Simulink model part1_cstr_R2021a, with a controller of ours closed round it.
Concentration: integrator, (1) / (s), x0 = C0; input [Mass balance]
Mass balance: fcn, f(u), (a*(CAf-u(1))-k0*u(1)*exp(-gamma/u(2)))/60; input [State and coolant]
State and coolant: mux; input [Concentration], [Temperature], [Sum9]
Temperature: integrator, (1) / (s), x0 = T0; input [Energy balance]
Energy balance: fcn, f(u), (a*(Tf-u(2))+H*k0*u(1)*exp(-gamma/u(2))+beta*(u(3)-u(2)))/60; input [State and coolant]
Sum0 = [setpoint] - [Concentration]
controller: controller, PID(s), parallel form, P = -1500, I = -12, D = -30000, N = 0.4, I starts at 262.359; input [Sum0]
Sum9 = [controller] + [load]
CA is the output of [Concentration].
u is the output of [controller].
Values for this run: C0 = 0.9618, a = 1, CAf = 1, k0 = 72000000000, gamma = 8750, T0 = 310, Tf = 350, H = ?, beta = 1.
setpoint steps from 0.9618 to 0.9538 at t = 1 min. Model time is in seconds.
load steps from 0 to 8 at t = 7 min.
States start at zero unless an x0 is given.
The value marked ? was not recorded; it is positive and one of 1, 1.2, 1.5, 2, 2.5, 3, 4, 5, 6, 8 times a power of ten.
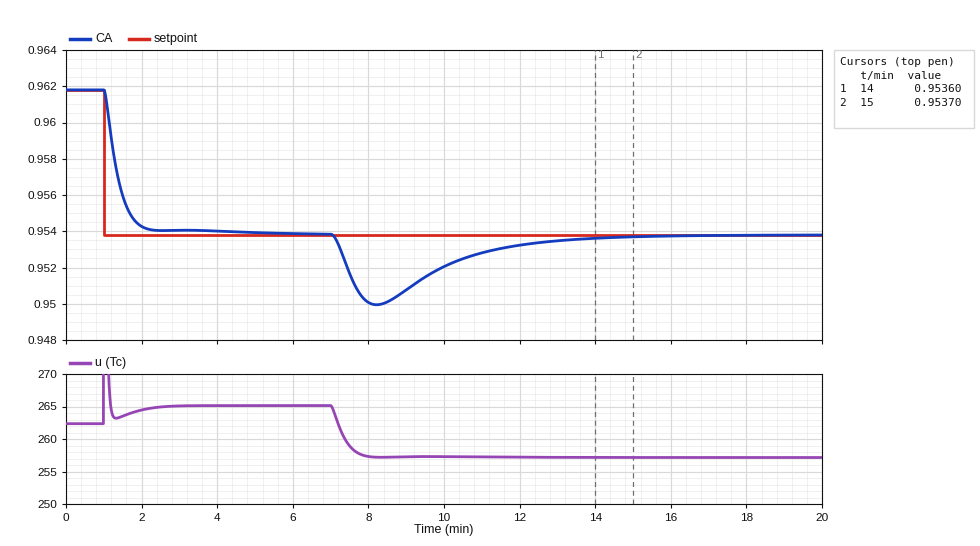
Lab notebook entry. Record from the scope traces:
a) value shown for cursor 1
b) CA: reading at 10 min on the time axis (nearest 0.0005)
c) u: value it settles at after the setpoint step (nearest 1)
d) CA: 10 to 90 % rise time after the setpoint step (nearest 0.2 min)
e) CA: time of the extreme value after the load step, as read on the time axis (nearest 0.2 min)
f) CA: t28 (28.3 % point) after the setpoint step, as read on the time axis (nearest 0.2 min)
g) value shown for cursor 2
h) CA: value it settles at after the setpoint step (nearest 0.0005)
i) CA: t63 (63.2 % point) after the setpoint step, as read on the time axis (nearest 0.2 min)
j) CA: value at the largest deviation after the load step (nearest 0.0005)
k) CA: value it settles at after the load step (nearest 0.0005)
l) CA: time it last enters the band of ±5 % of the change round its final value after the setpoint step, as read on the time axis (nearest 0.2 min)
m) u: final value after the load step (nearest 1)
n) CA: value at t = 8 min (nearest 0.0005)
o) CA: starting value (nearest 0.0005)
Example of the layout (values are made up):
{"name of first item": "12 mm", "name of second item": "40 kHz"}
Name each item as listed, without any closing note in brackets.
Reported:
{"value shown for cursor 1": "0.95360", "CA: reading at 10 min on the time axis": "0.9520", "u: value it settles at after the setpoint step": "265", "CA: 10 to 90 % rise time after the setpoint step": "0.8 min", "CA: time of the extreme value after the load step, as read on the time axis": "8.2 min", "CA: t28 (28.3 % point) after the setpoint step, as read on the time axis": "1.2 min", "value shown for cursor 2": "0.95370", "CA: value it settles at after the setpoint step": "0.9540", "CA: t63 (63.2 % point) after the setpoint step, as read on the time axis": "1.4 min", "CA: value at the largest deviation after the load step": "0.9500", "CA: value it settles at after the load step": "0.9540", "CA: time it last enters the band of ±5 % of the change round its final value after the setpoint step, as read on the time axis": "2.0 min", "u: final value after the load step": "257", "CA: value at t = 8 min": "0.9500", "CA: starting value": "0.9620"}
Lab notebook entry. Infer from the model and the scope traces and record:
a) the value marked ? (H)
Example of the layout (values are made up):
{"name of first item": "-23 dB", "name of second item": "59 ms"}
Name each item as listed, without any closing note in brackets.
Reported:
{"the value marked ?": "200"}
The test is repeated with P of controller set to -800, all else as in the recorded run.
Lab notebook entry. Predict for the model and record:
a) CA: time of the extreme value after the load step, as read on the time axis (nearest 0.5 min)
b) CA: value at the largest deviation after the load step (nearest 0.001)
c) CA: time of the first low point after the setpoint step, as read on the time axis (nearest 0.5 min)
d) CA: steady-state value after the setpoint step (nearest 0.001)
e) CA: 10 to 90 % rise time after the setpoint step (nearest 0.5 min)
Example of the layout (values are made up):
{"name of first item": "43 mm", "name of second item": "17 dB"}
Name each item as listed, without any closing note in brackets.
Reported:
{"CA: time of the extreme value after the load step, as read on the time axis": "8.5 min", "CA: value at the largest deviation after the load step": "0.949", "CA: time of the first low point after the setpoint step, as read on the time axis": "4.5 min", "CA: steady-state value after the setpoint step": "0.954", "CA: 10 to 90 % rise time after the setpoint step": "1.5 min"}
